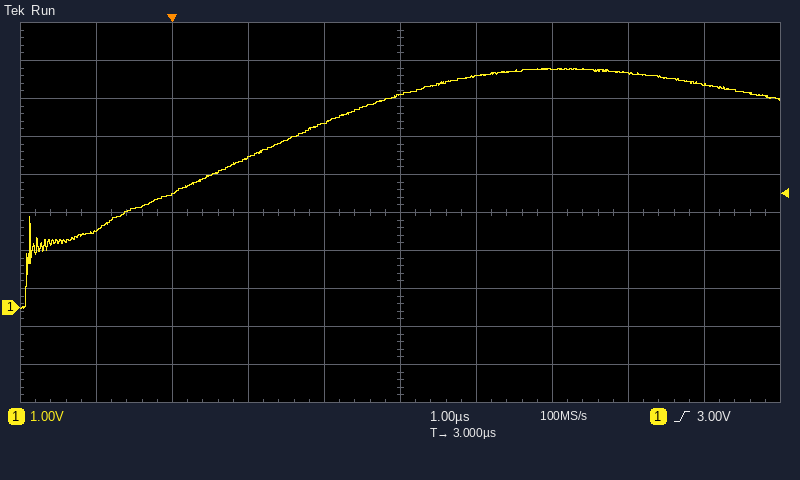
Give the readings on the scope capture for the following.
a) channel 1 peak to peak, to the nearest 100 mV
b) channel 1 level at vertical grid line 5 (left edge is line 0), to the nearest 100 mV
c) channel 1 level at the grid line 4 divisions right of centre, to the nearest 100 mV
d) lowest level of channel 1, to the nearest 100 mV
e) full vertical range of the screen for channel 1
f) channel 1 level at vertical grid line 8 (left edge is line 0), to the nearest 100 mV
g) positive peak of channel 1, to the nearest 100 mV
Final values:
6.3 V
5.6 V
5.9 V
0.0 V
10 V
6.2 V
6.3 V
